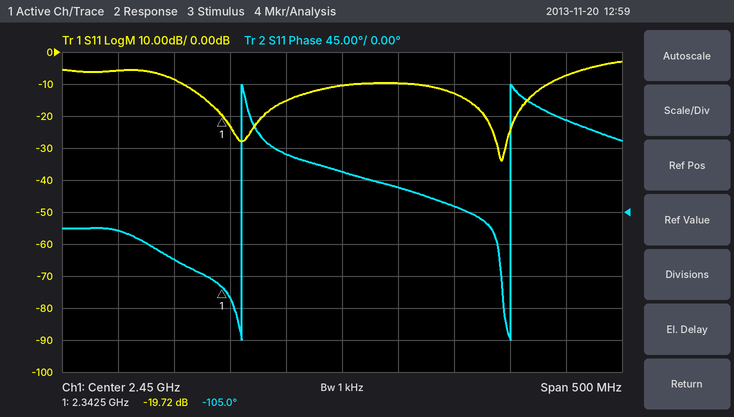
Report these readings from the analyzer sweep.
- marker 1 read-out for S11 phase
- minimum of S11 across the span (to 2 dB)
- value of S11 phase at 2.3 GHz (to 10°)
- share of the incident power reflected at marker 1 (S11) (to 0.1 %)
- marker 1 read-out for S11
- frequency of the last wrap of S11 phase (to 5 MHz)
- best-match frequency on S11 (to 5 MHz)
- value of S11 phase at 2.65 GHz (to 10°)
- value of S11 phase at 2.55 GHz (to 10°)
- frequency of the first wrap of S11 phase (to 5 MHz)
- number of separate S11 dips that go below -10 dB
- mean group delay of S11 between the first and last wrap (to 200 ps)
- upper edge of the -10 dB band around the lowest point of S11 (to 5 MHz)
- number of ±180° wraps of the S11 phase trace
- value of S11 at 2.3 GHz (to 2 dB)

-105.0°
-34 dB
-70°
1.1 %
-19.72 dB
2.600 GHz
2.590 GHz
130°
10°
2.360 GHz
2
4.2 ns
2.635 GHz
2
-8 dB
